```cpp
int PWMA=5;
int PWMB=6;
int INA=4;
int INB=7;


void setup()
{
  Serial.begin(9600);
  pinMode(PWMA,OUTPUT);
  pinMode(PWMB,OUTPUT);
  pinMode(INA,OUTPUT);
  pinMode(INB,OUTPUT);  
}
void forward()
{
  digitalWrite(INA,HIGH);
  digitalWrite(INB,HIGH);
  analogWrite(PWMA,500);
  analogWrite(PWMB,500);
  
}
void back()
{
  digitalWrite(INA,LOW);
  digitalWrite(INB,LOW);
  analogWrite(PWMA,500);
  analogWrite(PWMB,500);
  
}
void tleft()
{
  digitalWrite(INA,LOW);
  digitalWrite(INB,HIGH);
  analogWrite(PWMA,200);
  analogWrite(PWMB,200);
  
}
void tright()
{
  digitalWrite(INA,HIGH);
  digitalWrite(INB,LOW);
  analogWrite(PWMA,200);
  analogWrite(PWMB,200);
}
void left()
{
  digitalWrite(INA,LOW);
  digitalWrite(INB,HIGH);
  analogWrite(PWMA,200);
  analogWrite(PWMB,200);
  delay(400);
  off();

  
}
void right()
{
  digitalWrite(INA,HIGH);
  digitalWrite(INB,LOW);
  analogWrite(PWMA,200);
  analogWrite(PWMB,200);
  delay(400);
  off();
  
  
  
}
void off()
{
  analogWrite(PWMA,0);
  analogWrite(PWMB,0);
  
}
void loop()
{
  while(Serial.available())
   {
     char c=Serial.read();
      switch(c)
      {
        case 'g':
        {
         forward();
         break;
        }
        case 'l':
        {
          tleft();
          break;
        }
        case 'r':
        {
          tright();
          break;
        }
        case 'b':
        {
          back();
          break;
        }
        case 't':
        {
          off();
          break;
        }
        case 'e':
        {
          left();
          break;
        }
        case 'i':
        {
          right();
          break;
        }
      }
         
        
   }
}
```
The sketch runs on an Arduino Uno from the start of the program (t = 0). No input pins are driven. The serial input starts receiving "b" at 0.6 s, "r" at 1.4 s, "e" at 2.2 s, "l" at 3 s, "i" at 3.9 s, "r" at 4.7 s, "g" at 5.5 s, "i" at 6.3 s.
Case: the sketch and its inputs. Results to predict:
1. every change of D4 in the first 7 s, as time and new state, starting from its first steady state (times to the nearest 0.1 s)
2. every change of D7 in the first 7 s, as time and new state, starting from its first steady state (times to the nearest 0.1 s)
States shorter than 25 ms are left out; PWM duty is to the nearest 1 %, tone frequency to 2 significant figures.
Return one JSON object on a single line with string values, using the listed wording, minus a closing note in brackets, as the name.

{"every change of D4 in the first 7 s, as time and new state, starting from its first steady state": "0 s low; 1.4 s high; 2.2 s low; 3.9 s high", "every change of D7 in the first 7 s, as time and new state, starting from its first steady state": "0 s low; 2.2 s high; 3.9 s low; 5.5 s high; 6.3 s low"}
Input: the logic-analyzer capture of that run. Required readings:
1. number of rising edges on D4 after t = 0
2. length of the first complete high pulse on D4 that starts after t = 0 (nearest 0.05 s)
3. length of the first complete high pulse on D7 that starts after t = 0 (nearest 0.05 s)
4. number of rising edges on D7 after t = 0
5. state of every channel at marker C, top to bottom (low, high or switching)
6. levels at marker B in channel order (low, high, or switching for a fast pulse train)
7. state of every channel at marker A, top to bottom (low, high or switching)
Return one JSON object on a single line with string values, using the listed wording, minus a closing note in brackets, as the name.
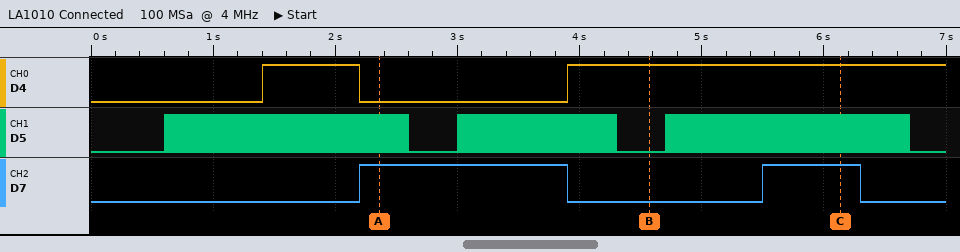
{"number of rising edges on D4 after t = 0": "2", "length of the first complete high pulse on D4 that starts after t = 0": "0.80 s", "length of the first complete high pulse on D7 that starts after t = 0": "1.70 s", "number of rising edges on D7 after t = 0": "2", "state of every channel at marker C, top to bottom": "D4 high, D5 switching, D7 high", "levels at marker B in channel order": "D4 high, D5 low, D7 low", "state of every channel at marker A, top to bottom": "D4 low, D5 switching, D7 high"}
